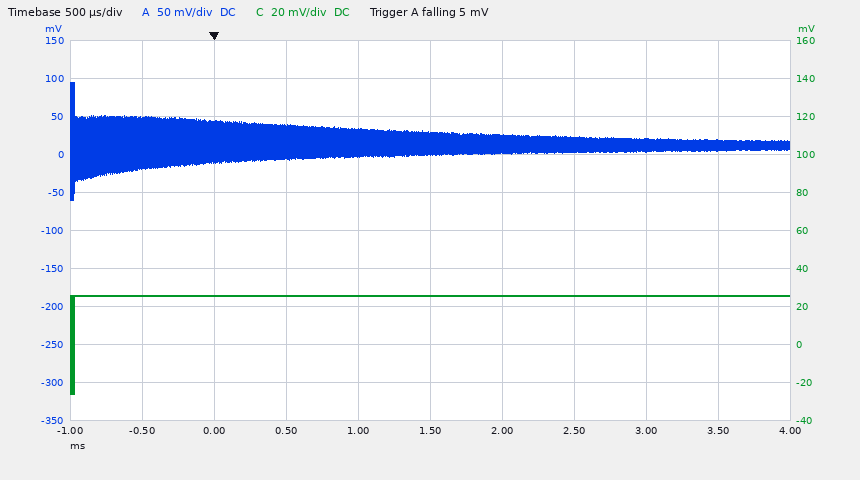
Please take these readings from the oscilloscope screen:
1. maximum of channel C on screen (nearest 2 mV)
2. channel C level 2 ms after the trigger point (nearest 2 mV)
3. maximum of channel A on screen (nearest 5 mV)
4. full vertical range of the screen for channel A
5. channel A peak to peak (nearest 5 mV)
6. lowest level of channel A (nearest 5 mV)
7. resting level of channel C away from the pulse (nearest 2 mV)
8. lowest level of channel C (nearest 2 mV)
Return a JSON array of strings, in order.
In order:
["26 mV", "26 mV", "95 mV", "500 mV", "155 mV", "-60 mV", "26 mV", "-26 mV"]
